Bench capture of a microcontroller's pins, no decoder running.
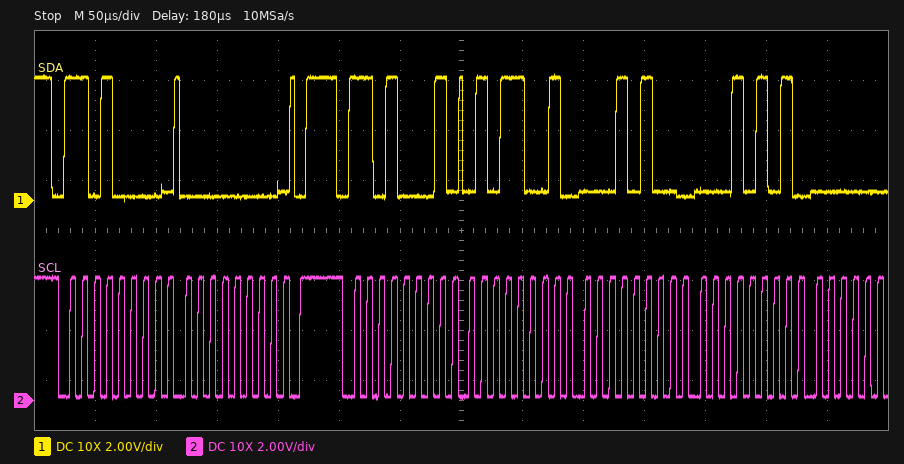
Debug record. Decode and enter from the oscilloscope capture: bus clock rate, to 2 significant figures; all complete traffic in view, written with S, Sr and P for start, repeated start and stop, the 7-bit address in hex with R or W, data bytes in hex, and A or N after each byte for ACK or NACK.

100 kHz
S 68W A 00 A P S 68R A 59 A 14 A 15 A
